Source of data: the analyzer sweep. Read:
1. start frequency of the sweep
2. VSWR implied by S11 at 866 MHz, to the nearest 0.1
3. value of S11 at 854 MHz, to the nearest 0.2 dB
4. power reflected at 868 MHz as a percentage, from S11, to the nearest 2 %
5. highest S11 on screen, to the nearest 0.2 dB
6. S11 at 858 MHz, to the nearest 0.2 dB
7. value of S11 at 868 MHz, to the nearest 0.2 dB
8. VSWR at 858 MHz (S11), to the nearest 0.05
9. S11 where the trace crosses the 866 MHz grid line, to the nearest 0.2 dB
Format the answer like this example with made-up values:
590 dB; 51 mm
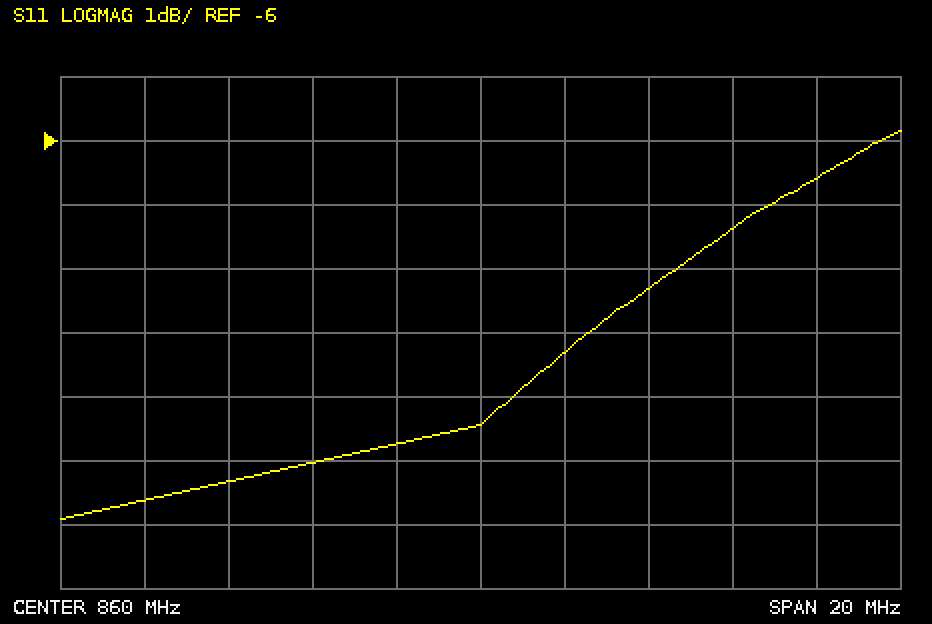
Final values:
850 MHz; 2.5; -11.4 dB; 22 %; -5.8 dB; -10.8 dB; -6.6 dB; 1.80; -7.4 dB
